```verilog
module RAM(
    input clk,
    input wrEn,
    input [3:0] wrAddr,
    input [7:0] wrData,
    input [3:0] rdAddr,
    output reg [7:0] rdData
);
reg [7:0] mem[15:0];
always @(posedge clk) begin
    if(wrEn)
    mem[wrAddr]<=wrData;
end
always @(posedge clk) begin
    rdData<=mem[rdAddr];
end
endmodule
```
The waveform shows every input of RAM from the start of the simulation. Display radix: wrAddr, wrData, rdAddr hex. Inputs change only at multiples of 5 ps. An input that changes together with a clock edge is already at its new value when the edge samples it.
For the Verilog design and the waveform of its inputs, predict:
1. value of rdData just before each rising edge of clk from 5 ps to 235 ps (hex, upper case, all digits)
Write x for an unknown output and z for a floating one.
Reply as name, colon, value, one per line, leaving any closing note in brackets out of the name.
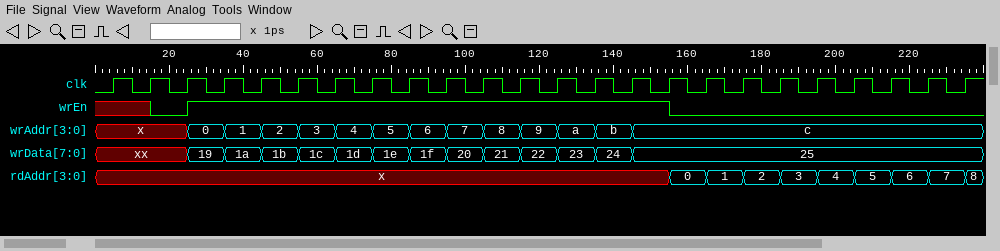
value of rdData just before each rising edge of clk from 5 ps to 235 ps: x, x, x, x, x, x, x, x, x, x, x, x, x, x, x, x, 19, 1A, 1B, 1C, 1D, 1E, 1F, 20
